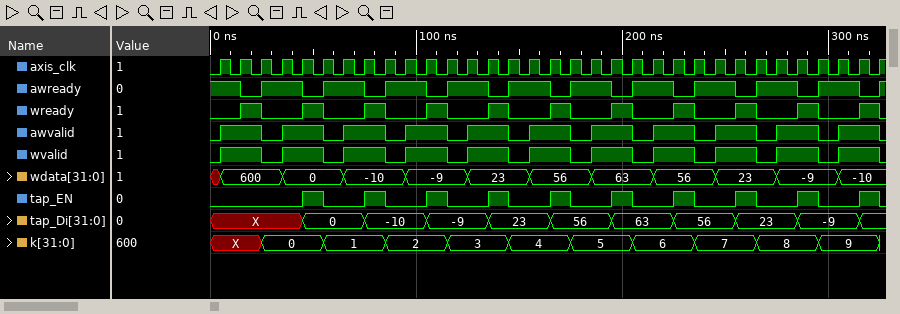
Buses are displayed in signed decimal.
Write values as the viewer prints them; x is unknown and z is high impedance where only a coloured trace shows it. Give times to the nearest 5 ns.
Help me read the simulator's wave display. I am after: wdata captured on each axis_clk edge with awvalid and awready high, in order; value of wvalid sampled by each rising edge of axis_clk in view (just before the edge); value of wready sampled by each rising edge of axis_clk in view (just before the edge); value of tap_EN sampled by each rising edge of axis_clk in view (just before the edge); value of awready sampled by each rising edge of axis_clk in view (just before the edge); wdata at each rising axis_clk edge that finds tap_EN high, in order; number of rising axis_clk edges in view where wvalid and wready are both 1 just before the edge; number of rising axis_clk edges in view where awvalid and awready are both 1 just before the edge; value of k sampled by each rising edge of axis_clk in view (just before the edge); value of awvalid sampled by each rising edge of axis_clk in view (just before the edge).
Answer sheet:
600, 0, -10, -9, 23, 56, 63, 56, 23, -9, -10
0 1 1 0 1 1 0 1 1 0 1 1 0 1 1 0 1 1 0 1 1 0 1 1 0 1 1 0 1 1 0 1 1
0 0 1 0 0 1 0 0 1 0 0 1 0 0 1 0 0 1 0 0 1 0 0 1 0 0 1 0 0 1 0 0 1
0 0 0 0 0 1 0 0 1 0 0 1 0 0 1 0 0 1 0 0 1 0 0 1 0 0 1 0 0 1 0 0 1
1 1 0 1 1 0 1 1 0 1 1 0 1 1 0 1 1 0 1 1 0 1 1 0 1 1 0 1 1 0 1 1 0
0, -10, -9, 23, 56, 63, 56, 23, -9, -10
11
11
X, X, X, 0, 0, 0, 1, 1, 1, 2, 2, 2, 3, 3, 3, 4, 4, 4, 5, 5, 5, 6, 6, 6, 7, 7, 7, 8, 8, 8, 9, 9, 9
0 1 1 0 1 1 0 1 1 0 1 1 0 1 1 0 1 1 0 1 1 0 1 1 0 1 1 0 1 1 0 1 1
